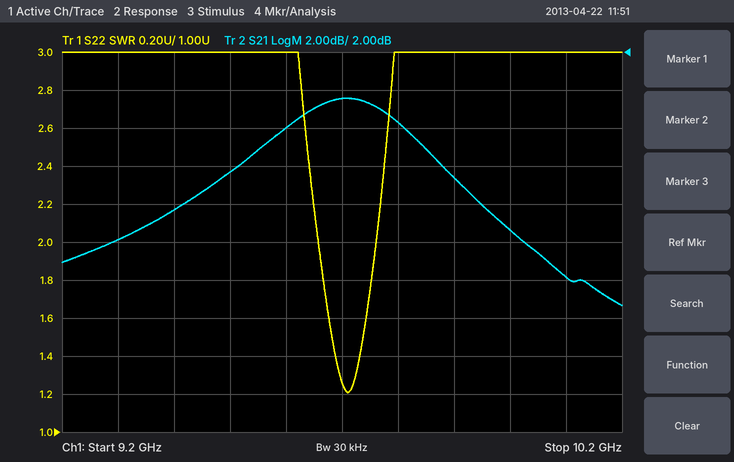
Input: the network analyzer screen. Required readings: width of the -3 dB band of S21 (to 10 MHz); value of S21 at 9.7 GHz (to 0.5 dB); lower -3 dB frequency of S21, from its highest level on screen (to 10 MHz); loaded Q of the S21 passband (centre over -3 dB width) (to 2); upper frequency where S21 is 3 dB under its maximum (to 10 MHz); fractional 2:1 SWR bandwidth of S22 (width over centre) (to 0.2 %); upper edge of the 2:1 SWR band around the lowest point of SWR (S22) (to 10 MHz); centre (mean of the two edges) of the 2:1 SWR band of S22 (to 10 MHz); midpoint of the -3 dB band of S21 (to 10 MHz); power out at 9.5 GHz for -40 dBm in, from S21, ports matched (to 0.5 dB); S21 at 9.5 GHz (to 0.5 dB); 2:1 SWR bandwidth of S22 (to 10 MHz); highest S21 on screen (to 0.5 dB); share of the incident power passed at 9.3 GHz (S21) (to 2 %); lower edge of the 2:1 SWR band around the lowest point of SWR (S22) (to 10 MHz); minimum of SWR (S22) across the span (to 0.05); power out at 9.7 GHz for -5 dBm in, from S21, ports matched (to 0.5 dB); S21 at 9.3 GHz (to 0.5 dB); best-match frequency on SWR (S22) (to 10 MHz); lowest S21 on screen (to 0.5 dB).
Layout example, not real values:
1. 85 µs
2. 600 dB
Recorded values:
1. 320 MHz
2. -0.5 dB
3. 9.54 GHz
4. 30
5. 9.86 GHz
6. 1.0 %
7. 9.76 GHz
8. 9.71 GHz
9. 9.70 GHz
10. -44.5 dBm
11. -4.5 dB
12. 100 MHz
13. -0.5 dB
14. 16 %
15. 9.66 GHz
16. 1.20
17. -5.5 dBm
18. -8.0 dB
19. 9.71 GHz
20. -11.5 dB
